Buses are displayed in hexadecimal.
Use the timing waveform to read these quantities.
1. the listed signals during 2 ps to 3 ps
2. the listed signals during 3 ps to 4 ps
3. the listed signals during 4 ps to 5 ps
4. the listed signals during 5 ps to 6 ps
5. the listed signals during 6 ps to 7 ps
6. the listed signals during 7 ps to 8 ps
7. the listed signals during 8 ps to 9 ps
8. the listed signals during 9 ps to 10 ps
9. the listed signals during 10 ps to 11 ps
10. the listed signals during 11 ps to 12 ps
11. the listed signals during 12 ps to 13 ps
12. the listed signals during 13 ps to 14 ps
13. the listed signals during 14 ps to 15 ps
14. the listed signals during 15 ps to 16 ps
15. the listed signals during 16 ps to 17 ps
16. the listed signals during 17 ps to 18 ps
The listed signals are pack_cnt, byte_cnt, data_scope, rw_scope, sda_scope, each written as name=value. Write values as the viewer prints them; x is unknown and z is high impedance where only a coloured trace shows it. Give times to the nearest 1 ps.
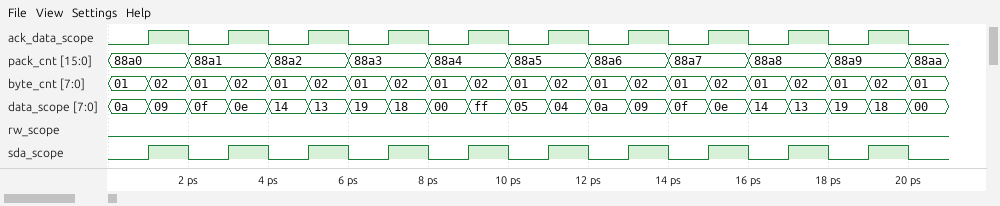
pack_cnt=88a1, byte_cnt=01, data_scope=0f, rw_scope=0, sda_scope=0
pack_cnt=88a1, byte_cnt=02, data_scope=0e, rw_scope=0, sda_scope=1
pack_cnt=88a2, byte_cnt=01, data_scope=14, rw_scope=0, sda_scope=0
pack_cnt=88a2, byte_cnt=02, data_scope=13, rw_scope=0, sda_scope=1
pack_cnt=88a3, byte_cnt=01, data_scope=19, rw_scope=0, sda_scope=0
pack_cnt=88a3, byte_cnt=02, data_scope=18, rw_scope=0, sda_scope=1
pack_cnt=88a4, byte_cnt=01, data_scope=00, rw_scope=0, sda_scope=0
pack_cnt=88a4, byte_cnt=02, data_scope=ff, rw_scope=0, sda_scope=1
pack_cnt=88a5, byte_cnt=01, data_scope=05, rw_scope=0, sda_scope=0
pack_cnt=88a5, byte_cnt=02, data_scope=04, rw_scope=0, sda_scope=1
pack_cnt=88a6, byte_cnt=01, data_scope=0a, rw_scope=0, sda_scope=0
pack_cnt=88a6, byte_cnt=02, data_scope=09, rw_scope=0, sda_scope=1
pack_cnt=88a7, byte_cnt=01, data_scope=0f, rw_scope=0, sda_scope=0
pack_cnt=88a7, byte_cnt=02, data_scope=0e, rw_scope=0, sda_scope=1
pack_cnt=88a8, byte_cnt=01, data_scope=14, rw_scope=0, sda_scope=0
pack_cnt=88a8, byte_cnt=02, data_scope=13, rw_scope=0, sda_scope=1
